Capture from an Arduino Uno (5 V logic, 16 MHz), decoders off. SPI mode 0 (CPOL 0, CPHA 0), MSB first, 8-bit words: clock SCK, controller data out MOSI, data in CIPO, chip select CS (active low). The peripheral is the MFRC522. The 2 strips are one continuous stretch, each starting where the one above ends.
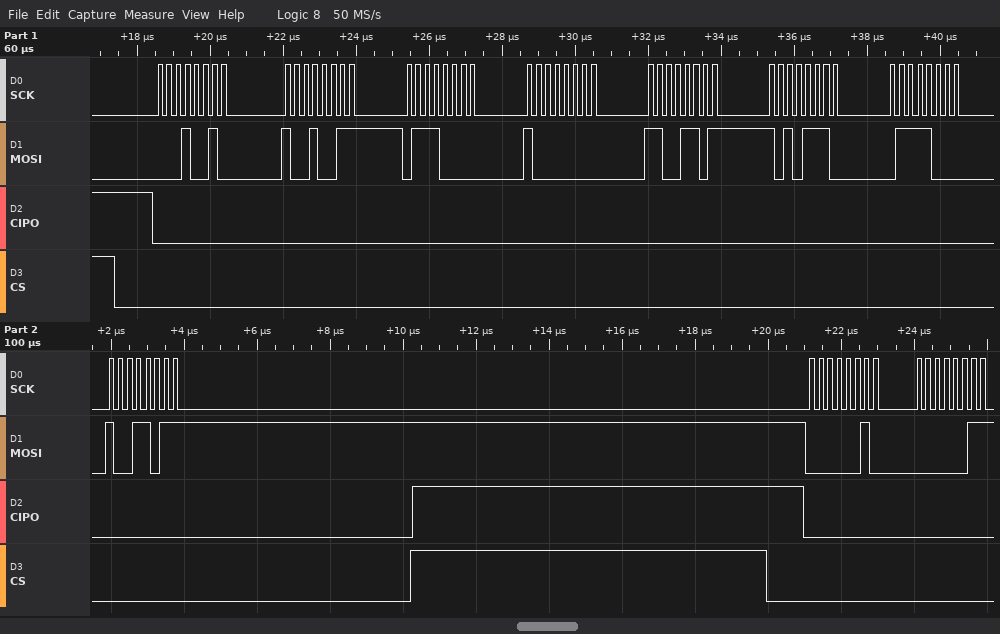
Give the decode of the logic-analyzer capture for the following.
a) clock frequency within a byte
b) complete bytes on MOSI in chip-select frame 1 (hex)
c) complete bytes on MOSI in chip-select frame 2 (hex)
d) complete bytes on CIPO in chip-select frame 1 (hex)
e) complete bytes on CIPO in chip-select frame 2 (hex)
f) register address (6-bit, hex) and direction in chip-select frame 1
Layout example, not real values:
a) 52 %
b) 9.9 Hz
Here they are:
a) 4 MHz
b) 12 93 70 80 CD AE 78 9B
c) 02 03
d) 00 00 00 00 00 00 00 00
e) 00 00
f) 0x09 write
